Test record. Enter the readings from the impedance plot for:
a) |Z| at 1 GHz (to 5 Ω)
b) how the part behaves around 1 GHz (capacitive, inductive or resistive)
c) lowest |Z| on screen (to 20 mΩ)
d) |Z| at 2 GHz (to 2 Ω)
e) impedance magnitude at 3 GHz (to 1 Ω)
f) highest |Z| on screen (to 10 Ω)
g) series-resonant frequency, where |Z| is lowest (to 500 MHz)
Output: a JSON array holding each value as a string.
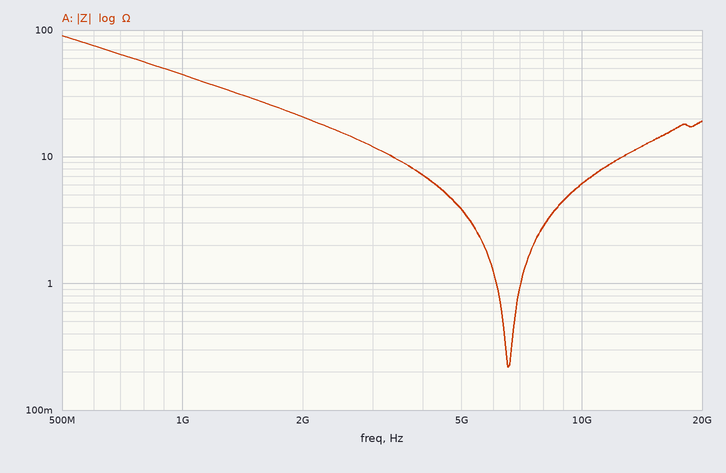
["45 Ω", "capacitive", "220 mΩ", "20 Ω", "12 Ω", "90 Ω", "6.5 GHz"]
